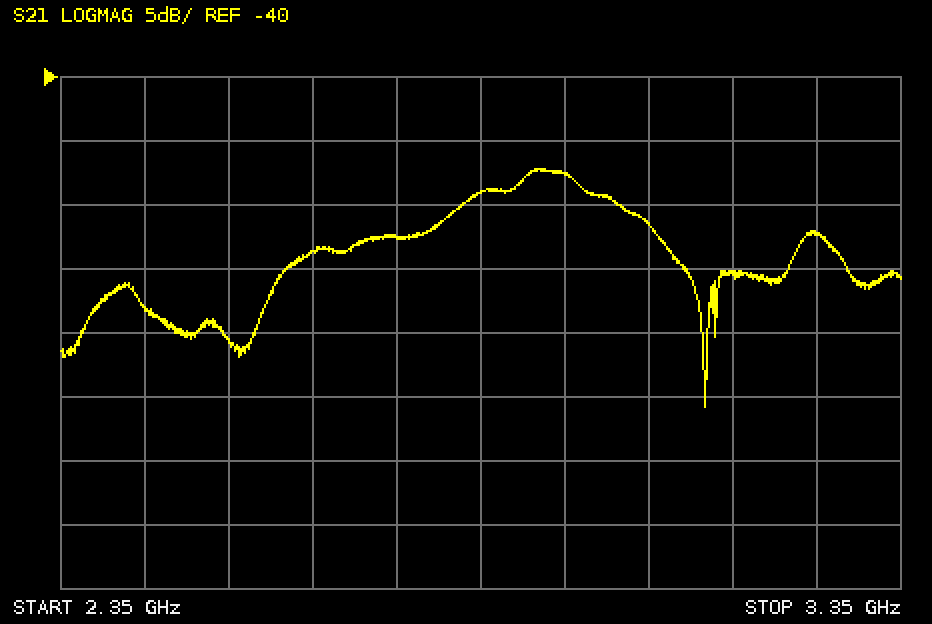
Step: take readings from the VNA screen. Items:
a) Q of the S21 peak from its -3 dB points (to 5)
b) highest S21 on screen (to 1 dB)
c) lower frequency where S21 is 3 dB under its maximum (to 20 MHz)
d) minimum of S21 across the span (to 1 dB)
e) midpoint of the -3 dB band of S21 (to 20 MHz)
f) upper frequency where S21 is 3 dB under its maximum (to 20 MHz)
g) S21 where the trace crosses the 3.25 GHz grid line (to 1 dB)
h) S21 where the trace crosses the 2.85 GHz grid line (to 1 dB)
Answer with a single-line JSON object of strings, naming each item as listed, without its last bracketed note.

{"Q of the S21 peak from its -3 dB points": "15", "highest S21 on screen": "-47 dB", "lower frequency where S21 is 3 dB under its maximum": "2.82 GHz", "minimum of S21 across the span": "-66 dB", "midpoint of the -3 dB band of S21": "2.92 GHz", "upper frequency where S21 is 3 dB under its maximum": "3.02 GHz", "S21 where the trace crosses the 3.25 GHz grid line": "-52 dB", "S21 where the trace crosses the 2.85 GHz grid line": "-49 dB"}
